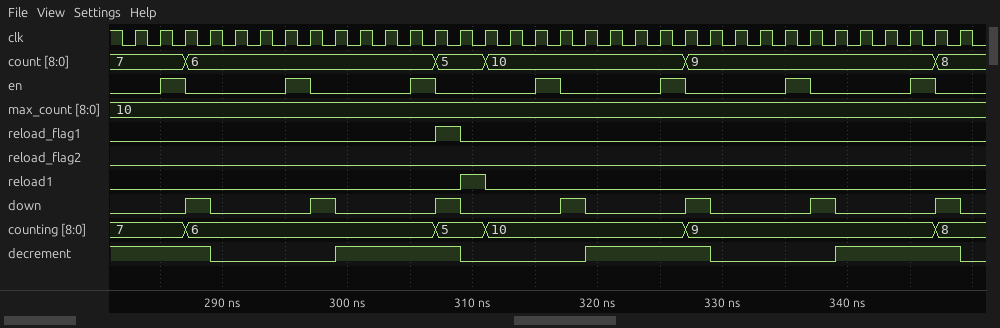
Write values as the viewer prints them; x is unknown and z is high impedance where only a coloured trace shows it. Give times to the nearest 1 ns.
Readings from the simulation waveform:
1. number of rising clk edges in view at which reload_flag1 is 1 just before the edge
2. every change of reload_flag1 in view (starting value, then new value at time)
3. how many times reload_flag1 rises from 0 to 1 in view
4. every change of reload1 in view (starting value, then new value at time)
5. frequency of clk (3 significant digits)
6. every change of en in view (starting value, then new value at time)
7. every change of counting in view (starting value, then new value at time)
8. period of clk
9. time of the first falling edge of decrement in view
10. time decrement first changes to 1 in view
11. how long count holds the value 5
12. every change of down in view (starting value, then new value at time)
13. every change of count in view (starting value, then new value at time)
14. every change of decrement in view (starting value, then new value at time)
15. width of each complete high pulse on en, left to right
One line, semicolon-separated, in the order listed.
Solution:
1; 0, 1 at 307 ns, 0 at 309 ns; 1; 0, 1 at 309 ns, 0 at 311 ns; 500 MHz; 0, 1 at 285 ns, 0 at 287 ns, 1 at 295 ns, 0 at 297 ns, 1 at 305 ns, 0 at 307 ns, 1 at 315 ns, 0 at 317 ns, 1 at 325 ns, 0 at 327 ns, 1 at 335 ns, 0 at 337 ns, 1 at 345 ns, 0 at 347 ns; 7, 6 at 287 ns, 5 at 307 ns, 10 at 311 ns, 9 at 327 ns, 8 at 347 ns; 2 ns; 289 ns; 299 ns; 4 ns; 0, 1 at 287 ns, 0 at 289 ns, 1 at 297 ns, 0 at 299 ns, 1 at 307 ns, 0 at 309 ns, 1 at 317 ns, 0 at 319 ns, 1 at 327 ns, 0 at 329 ns, 1 at 337 ns, 0 at 339 ns, 1 at 347 ns, 0 at 349 ns; 7, 6 at 287 ns, 5 at 307 ns, 10 at 311 ns, 9 at 327 ns, 8 at 347 ns; 1, 0 at 289 ns, 1 at 299 ns, 0 at 309 ns, 1 at 319 ns, 0 at 329 ns, 1 at 339 ns, 0 at 349 ns; 2 ns, 2 ns, 2 ns, 2 ns, 2 ns, 2 ns, 2 ns
